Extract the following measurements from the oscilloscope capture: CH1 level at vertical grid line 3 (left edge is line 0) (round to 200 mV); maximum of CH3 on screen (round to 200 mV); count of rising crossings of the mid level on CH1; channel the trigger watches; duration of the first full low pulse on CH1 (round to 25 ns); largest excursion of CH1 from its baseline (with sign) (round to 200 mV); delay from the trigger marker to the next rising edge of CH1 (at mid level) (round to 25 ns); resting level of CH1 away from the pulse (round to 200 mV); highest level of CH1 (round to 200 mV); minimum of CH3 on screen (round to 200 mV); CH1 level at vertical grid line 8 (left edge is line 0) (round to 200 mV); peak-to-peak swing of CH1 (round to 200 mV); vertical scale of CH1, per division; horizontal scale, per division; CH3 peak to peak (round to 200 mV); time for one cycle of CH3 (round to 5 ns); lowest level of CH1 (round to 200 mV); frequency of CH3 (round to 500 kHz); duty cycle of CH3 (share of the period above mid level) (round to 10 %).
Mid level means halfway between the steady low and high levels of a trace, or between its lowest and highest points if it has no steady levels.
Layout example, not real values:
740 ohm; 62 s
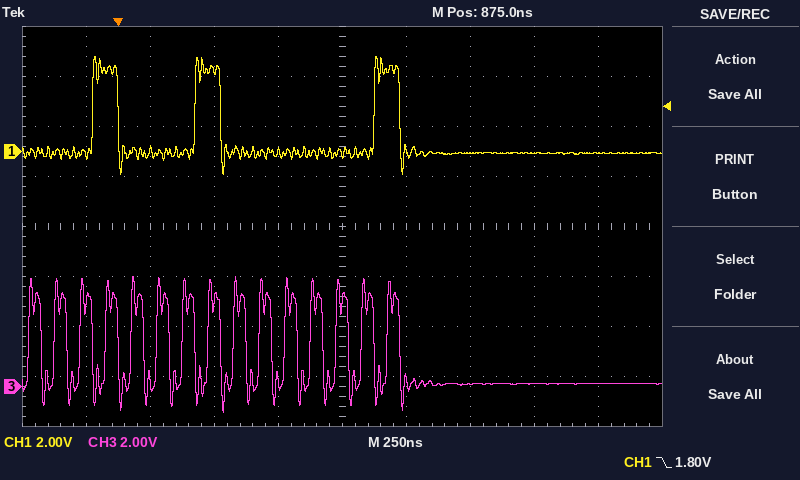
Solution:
3.2 V; 4.4 V; 3; CH1; 300 ns; +3.8 V; 300 ns; 0.0 V; 3.8 V; -1.0 V; 0.0 V; 4.8 V; 2 V; 250 ns; 5.4 V; 100 ns; -1.0 V; 10.0 MHz; 50 %
